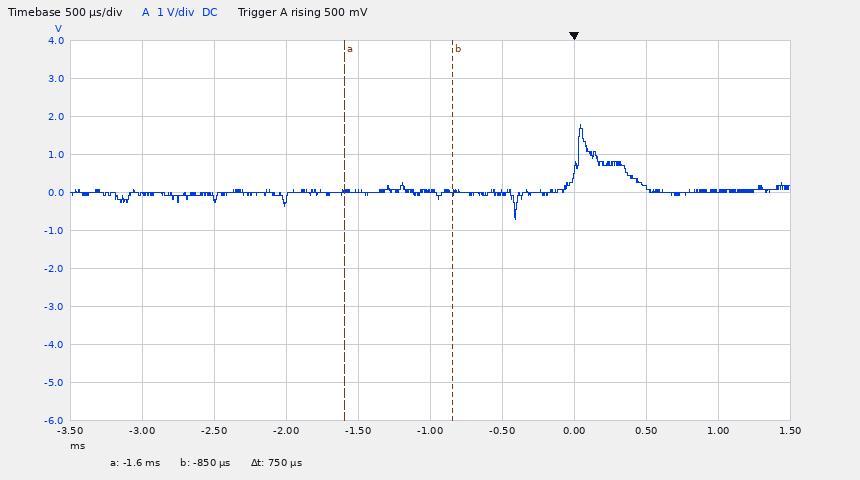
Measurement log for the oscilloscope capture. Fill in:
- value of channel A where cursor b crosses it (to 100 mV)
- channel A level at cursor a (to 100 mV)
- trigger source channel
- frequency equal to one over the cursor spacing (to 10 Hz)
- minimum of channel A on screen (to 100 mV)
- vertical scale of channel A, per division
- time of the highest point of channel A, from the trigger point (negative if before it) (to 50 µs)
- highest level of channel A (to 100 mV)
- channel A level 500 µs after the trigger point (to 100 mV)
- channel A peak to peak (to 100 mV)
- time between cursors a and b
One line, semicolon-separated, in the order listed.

0.0 V; 0.0 V; channel A; 1.33 kHz; -700 mV; 1 V; +50 µs; 1.8 V; 100 mV; 2.5 V; 750 µs
